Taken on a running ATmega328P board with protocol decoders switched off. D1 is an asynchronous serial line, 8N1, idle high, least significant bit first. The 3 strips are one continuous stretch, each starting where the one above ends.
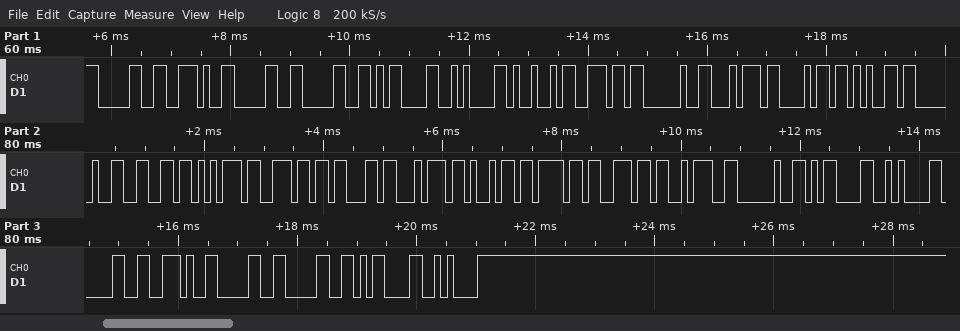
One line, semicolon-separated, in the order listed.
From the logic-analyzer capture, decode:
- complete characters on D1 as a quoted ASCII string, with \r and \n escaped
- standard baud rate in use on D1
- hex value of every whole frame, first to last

"0.00\r\nIn the function: \r\n0.00\r\n"; 9600 baud; 30 2E 30 30 0D 0A 49 6E 20 74 68 65 20 66 75 6E 63 74 69 6F 6E 3A 20 0D 0A 30 2E 30 30 0D 0A
